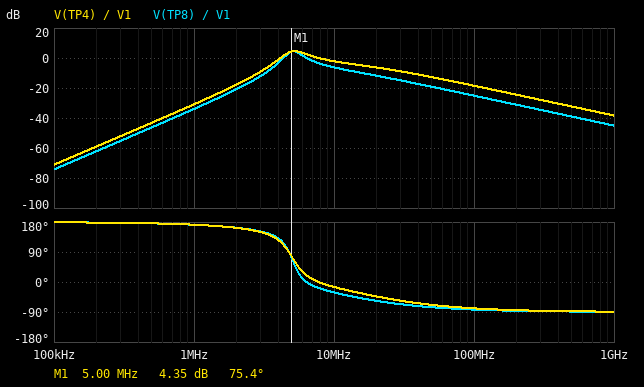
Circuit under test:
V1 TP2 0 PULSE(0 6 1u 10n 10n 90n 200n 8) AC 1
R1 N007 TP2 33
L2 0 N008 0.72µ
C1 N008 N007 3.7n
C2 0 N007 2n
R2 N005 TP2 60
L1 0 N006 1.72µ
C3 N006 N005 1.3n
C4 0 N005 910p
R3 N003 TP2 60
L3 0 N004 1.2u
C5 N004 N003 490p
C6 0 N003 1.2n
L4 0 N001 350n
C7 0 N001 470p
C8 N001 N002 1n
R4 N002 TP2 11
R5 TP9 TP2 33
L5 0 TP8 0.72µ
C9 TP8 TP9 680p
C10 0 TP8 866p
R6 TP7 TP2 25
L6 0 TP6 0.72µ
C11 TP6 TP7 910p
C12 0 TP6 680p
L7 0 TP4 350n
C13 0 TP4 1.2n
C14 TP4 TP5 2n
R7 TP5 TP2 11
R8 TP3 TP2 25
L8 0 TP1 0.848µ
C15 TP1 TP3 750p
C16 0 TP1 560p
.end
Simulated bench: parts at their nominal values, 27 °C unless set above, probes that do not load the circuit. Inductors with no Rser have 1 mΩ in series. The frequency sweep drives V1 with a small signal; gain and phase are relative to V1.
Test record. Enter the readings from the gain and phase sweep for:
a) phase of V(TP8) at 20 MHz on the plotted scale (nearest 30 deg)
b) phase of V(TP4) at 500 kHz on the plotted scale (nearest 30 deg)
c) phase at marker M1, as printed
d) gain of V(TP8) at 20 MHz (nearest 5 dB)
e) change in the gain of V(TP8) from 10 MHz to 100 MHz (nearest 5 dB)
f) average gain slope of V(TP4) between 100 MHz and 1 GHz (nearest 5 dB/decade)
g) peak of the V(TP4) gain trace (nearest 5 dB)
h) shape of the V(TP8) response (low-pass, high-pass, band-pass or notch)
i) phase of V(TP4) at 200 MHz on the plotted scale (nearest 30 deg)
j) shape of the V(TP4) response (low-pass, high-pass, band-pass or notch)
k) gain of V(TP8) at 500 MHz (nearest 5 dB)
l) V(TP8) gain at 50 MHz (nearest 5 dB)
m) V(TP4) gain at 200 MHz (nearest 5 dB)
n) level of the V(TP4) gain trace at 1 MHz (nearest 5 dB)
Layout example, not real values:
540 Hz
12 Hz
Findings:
-60 deg
180 deg
75.4 deg
-10 dB
-20 dB
-20 dB/decade
5 dB
band-pass
-90 deg
band-pass
-40 dB
-20 dB
-25 dB
-30 dB
